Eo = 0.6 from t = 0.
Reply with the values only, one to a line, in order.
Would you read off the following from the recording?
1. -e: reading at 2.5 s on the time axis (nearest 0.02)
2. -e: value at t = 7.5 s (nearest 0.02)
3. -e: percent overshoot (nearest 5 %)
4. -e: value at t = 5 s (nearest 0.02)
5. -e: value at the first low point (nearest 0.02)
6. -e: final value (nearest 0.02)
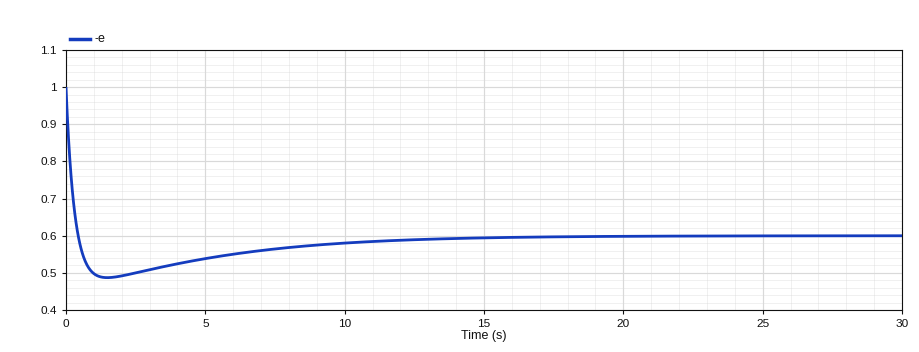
0.50
0.56
30 %
0.54
0.48
0.60
